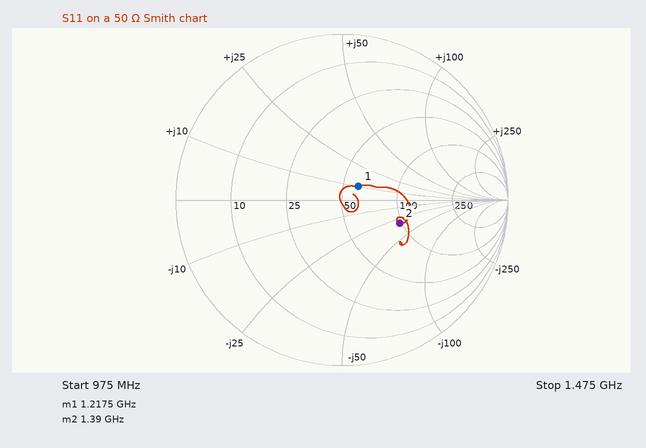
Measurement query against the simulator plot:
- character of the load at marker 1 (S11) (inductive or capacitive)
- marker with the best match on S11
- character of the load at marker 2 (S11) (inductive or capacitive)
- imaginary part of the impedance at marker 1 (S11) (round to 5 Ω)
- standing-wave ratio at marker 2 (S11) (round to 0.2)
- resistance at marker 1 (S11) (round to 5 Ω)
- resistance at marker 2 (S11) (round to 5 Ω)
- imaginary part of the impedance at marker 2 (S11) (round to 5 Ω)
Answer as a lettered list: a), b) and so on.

a) inductive
b) marker 1
c) capacitive
d) +10 Ω
e) 2.2
f) 60 Ω
g) 95 Ω
h) -30 Ω
